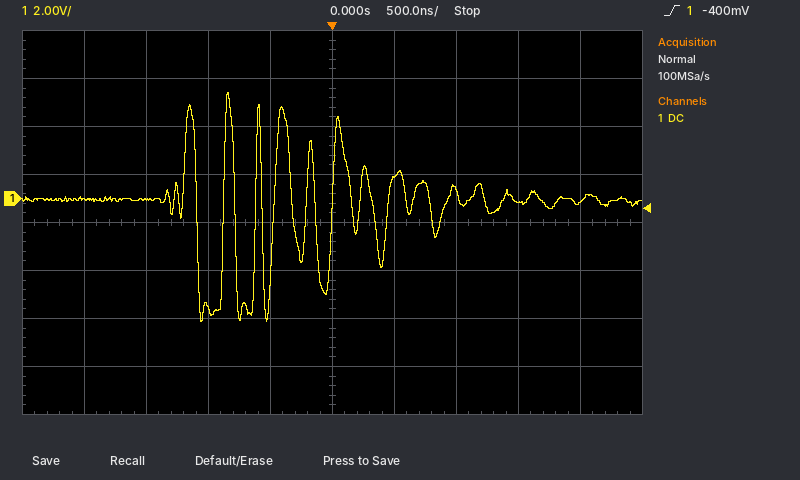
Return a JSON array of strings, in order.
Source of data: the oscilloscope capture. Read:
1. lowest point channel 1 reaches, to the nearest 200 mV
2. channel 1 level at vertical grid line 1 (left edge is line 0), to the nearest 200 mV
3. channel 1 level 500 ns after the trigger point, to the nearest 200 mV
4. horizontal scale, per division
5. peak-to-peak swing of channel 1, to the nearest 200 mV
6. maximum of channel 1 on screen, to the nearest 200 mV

["-5.2 V", "0.0 V", "800 mV", "500 ns", "9.6 V", "4.4 V"]
